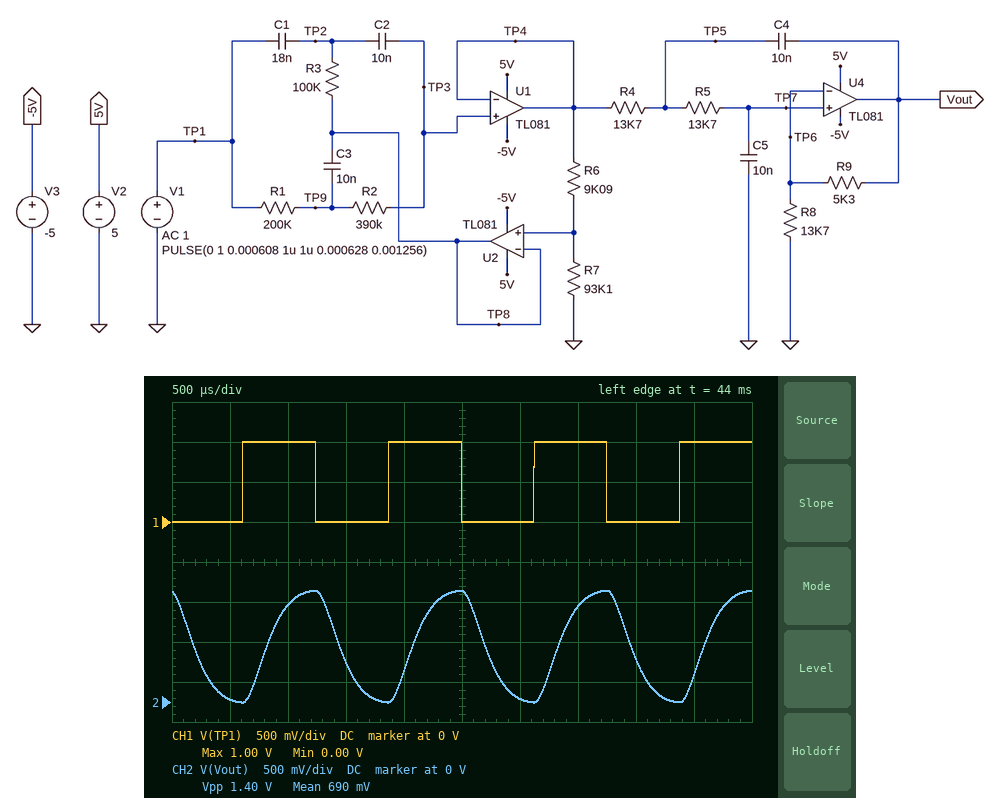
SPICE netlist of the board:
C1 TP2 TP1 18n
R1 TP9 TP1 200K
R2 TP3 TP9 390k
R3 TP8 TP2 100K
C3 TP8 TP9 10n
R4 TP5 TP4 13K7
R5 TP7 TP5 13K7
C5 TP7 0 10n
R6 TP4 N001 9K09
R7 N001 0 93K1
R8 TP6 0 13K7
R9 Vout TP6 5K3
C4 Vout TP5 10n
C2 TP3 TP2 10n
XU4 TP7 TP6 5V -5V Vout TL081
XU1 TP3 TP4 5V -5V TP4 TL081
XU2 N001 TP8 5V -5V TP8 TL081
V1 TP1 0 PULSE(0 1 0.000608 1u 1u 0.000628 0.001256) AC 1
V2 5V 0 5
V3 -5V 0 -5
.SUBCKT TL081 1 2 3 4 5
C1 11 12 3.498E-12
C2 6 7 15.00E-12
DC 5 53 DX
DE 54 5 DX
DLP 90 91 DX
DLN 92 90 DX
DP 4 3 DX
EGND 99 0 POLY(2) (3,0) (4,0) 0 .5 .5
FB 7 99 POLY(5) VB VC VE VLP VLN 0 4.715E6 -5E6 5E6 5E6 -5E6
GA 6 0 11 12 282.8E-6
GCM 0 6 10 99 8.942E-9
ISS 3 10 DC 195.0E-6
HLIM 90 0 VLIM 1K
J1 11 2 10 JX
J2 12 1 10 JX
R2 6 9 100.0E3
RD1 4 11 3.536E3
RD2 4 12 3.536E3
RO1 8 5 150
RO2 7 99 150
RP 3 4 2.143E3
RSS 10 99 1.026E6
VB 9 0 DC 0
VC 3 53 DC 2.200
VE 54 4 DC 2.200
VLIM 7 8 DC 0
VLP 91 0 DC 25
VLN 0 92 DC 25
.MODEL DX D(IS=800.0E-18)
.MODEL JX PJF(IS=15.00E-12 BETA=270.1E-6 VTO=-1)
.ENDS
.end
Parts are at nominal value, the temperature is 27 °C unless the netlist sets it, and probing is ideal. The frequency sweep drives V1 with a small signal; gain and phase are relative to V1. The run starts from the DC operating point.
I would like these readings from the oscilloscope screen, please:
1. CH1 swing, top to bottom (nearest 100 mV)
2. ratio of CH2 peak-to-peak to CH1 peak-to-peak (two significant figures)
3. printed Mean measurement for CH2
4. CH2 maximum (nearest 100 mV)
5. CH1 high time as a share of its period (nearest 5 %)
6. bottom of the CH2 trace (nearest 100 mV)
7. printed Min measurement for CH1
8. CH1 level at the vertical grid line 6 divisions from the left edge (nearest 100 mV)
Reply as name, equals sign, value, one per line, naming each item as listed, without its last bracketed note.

CH1 swing, top to bottom = 1.0 V
ratio of CH2 peak-to-peak to CH1 peak-to-peak = 1.4
printed Mean measurement for CH2 = 690 mV
CH2 maximum = 1.4 V
CH1 high time as a share of its period = 50 %
bottom of the CH2 trace = 0 V
printed Min measurement for CH1 = 0.00 V
CH1 level at the vertical grid line 6 divisions from the left edge = 0 V
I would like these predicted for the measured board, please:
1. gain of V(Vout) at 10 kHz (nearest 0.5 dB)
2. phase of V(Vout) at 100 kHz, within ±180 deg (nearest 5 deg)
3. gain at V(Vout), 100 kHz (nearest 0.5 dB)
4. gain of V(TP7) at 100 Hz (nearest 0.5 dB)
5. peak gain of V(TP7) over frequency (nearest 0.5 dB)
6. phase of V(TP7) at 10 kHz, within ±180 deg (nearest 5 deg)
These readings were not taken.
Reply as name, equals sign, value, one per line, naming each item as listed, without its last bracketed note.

gain of V(Vout) at 10 kHz = -34.5 dB
phase of V(Vout) at 100 kHz, within ±180 deg = 110 deg
gain at V(Vout), 100 kHz = -66.5 dB
gain of V(TP7) at 100 Hz = -0.5 dB
peak gain of V(TP7) over frequency = 0 dB
phase of V(TP7) at 10 kHz, within ±180 deg = -170 deg
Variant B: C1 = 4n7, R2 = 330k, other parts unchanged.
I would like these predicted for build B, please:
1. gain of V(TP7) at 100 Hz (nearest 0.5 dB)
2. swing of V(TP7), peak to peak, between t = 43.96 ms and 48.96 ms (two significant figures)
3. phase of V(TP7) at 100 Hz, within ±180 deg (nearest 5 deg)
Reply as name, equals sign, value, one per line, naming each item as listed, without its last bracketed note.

gain of V(TP7) at 100 Hz = -12.5 dB
swing of V(TP7), peak to peak, between t = 43.96 ms and 48.96 ms = 990 mV
phase of V(TP7) at 100 Hz, within ±180 deg = -45 deg
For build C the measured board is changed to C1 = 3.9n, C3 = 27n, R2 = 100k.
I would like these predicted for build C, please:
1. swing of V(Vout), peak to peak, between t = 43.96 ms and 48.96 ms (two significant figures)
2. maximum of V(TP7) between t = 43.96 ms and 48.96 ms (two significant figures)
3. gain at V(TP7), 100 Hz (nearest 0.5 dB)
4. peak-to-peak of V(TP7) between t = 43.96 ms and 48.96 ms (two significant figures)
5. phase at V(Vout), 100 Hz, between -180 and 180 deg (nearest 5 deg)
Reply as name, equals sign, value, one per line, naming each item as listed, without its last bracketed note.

swing of V(Vout), peak to peak, between t = 43.96 ms and 48.96 ms = 1.3 V
maximum of V(TP7) between t = 43.96 ms and 48.96 ms = 980 mV
gain at V(TP7), 100 Hz = -2.0 dB
peak-to-peak of V(TP7) between t = 43.96 ms and 48.96 ms = 970 mV
phase at V(Vout), 100 Hz, between -180 and 180 deg = -60 deg
